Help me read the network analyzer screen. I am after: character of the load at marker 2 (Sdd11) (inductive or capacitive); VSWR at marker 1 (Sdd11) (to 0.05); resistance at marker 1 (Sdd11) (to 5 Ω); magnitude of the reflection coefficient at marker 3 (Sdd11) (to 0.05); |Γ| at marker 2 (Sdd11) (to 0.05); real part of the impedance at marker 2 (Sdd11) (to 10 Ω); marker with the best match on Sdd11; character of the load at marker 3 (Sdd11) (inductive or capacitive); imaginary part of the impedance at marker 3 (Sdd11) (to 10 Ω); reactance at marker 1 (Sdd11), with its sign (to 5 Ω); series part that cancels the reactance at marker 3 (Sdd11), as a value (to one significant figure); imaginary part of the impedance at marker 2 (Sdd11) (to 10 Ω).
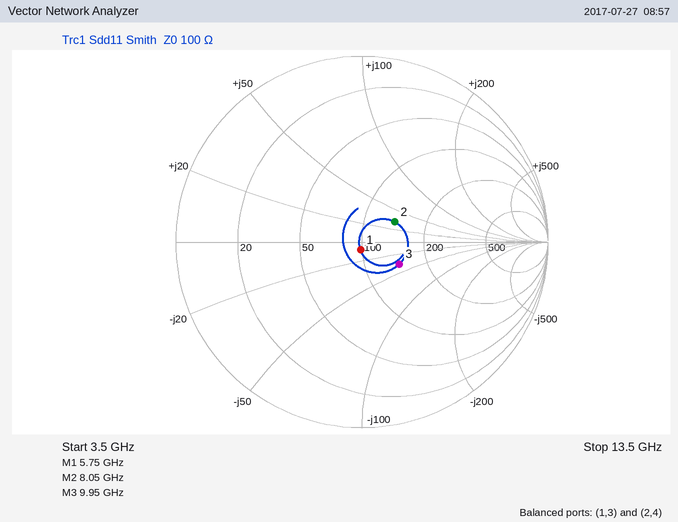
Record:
inductive
1.10
100 Ω
0.25
0.20
140 Ω
marker 1
capacitive
-40 Ω
-10 Ω
600 pH
+30 Ω
